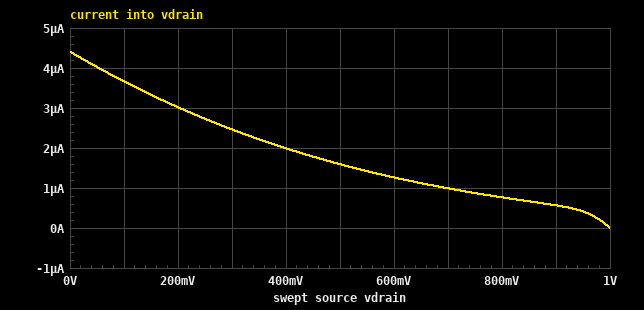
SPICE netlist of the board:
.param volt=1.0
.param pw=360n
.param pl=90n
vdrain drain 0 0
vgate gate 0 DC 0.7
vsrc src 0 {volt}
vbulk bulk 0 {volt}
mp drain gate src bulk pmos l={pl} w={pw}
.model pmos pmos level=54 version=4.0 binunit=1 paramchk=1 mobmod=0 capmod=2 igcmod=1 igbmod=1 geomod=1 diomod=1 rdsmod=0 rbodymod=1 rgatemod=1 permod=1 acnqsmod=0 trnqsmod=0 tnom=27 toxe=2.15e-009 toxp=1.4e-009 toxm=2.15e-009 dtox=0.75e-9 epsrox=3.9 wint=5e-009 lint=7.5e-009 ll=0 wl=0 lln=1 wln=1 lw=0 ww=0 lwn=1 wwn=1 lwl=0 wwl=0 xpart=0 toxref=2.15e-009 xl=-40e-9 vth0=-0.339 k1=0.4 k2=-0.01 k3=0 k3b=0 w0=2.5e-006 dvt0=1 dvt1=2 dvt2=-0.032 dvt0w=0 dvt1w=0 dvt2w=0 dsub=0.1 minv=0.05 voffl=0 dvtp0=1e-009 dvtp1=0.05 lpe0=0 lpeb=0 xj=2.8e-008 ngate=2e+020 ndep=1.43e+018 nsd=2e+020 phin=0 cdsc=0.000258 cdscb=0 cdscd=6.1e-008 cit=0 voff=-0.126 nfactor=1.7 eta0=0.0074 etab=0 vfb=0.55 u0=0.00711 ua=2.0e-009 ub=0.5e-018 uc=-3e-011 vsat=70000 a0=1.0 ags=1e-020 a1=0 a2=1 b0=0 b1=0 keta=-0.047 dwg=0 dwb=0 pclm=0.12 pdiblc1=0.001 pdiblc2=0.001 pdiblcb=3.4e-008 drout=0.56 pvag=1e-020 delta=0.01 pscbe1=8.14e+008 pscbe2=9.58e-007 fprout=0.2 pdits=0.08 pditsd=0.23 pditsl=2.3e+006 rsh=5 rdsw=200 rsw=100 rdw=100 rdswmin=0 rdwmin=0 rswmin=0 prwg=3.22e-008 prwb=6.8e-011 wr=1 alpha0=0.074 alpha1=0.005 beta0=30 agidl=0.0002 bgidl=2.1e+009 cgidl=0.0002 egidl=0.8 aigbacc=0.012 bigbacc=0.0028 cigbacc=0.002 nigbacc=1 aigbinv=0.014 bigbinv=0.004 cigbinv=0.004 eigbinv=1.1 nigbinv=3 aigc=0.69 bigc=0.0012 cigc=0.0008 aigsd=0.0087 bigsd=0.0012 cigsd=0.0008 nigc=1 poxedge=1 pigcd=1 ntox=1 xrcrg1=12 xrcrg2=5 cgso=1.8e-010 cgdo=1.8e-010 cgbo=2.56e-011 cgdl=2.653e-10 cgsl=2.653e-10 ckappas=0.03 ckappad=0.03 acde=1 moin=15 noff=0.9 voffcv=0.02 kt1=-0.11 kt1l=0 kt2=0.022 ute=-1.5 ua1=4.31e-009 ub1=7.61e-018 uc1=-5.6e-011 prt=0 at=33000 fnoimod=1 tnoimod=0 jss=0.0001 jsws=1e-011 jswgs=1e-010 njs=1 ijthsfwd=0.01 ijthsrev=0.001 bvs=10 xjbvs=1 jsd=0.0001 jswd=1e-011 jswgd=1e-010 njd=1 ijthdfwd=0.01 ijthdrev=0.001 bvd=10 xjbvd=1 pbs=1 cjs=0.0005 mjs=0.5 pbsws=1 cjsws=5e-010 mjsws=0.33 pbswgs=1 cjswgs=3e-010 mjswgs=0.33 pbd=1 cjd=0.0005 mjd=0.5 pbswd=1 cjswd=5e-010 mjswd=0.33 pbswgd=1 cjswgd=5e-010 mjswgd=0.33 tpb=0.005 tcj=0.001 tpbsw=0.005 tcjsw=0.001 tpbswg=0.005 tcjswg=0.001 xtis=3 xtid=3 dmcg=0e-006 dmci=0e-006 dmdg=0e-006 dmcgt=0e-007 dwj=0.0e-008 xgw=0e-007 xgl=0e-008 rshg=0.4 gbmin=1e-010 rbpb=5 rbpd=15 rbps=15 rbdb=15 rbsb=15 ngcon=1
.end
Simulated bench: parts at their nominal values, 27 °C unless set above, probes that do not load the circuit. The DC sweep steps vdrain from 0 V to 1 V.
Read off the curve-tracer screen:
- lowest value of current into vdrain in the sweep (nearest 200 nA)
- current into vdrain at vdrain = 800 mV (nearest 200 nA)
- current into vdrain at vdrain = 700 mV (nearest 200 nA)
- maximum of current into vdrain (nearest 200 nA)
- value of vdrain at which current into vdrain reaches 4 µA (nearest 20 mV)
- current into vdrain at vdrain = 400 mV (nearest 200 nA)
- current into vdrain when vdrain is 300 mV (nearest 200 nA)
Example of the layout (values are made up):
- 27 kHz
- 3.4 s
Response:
- 0 A
- 800 nA
- 1.0 µA
- 4.4 µA
- 60 mV
- 2.0 µA
- 2.4 µA
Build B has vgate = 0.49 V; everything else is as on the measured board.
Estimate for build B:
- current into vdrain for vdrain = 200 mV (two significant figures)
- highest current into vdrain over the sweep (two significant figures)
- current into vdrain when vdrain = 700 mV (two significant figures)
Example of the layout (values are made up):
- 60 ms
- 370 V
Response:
- 25 µA
- 30 µA
- 15 µA
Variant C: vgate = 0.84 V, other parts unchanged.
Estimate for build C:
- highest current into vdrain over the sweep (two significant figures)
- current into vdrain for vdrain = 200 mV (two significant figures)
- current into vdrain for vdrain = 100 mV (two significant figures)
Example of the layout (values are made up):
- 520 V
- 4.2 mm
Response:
- 320 nA
- 190 nA
- 250 nA
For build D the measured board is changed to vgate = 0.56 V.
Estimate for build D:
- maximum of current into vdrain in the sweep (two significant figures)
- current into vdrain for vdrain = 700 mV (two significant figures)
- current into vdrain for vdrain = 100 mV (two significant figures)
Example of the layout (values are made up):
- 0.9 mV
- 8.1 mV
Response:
- 19 µA
- 8.1 µA
- 17 µA
